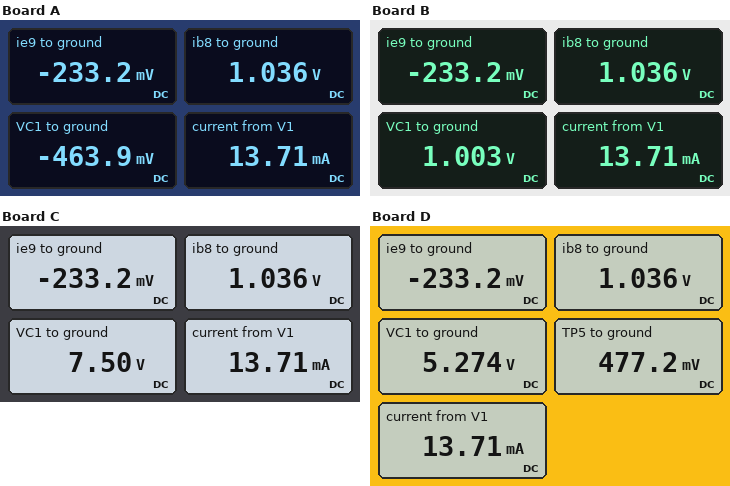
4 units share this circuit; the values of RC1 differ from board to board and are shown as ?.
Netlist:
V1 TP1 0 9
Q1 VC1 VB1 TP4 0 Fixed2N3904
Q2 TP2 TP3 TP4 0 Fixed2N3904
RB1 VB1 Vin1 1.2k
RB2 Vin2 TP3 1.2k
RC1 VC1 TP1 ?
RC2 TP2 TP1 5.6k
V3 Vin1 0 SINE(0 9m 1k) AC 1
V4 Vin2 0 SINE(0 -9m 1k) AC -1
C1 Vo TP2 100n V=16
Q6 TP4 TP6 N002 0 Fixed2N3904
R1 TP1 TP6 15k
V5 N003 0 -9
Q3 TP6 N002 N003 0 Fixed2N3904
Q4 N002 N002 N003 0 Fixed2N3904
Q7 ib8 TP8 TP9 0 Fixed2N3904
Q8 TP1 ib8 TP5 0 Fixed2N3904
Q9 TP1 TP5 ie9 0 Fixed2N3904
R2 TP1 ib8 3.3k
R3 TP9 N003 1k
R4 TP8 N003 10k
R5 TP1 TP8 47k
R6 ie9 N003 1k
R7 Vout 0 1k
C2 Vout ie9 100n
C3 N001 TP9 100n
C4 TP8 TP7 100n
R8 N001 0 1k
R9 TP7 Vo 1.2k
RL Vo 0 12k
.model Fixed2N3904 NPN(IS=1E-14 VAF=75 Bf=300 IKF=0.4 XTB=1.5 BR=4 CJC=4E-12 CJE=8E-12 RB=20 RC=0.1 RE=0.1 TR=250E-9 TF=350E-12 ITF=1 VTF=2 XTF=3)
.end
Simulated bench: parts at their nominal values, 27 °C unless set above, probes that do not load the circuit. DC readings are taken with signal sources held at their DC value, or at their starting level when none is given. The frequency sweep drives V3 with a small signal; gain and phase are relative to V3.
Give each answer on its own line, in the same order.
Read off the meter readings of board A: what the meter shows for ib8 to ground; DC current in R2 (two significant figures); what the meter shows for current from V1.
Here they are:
1.036 V
2.4 mA
13.71 mA
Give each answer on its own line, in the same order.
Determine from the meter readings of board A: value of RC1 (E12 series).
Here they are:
18 kΩ
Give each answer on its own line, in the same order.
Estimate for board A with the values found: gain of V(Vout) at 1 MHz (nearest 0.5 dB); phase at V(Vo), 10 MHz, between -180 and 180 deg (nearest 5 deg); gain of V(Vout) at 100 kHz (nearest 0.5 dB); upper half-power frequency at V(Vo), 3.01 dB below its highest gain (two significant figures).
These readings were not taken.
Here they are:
28.5 dB
-40 deg
40.5 dB
160 kHz
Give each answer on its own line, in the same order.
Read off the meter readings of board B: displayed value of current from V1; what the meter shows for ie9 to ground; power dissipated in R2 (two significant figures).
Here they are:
13.71 mA
-233.2 mV
19 mW
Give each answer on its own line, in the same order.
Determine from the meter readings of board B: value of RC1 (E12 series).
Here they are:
15 kΩ
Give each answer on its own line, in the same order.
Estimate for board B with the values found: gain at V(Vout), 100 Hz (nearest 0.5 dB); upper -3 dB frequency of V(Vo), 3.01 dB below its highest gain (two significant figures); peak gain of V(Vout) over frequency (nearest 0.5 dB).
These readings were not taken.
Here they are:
10.0 dB
250 kHz
48.5 dB
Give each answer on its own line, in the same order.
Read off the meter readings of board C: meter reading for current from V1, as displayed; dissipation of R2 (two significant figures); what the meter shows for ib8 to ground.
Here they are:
13.71 mA
19 mW
1.036 V
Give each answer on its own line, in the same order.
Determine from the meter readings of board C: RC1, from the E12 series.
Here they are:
2.7 kΩ
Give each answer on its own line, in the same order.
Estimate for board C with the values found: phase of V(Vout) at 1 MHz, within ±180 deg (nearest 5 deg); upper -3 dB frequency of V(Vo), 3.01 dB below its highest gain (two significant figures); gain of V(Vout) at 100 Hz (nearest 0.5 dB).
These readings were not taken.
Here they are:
120 deg
940 kHz
10.5 dB
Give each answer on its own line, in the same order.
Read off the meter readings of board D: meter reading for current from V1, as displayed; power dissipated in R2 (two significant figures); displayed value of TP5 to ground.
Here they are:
13.71 mA
19 mW
477.2 mV
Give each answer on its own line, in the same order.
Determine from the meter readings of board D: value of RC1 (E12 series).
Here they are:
6.8 kΩ
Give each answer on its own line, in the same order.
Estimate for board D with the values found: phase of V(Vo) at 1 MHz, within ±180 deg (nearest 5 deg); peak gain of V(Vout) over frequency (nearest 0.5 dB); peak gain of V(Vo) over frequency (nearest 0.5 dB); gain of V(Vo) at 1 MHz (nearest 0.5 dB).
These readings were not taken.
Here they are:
-65 deg
49.0 dB
34.0 dB
28.0 dB
